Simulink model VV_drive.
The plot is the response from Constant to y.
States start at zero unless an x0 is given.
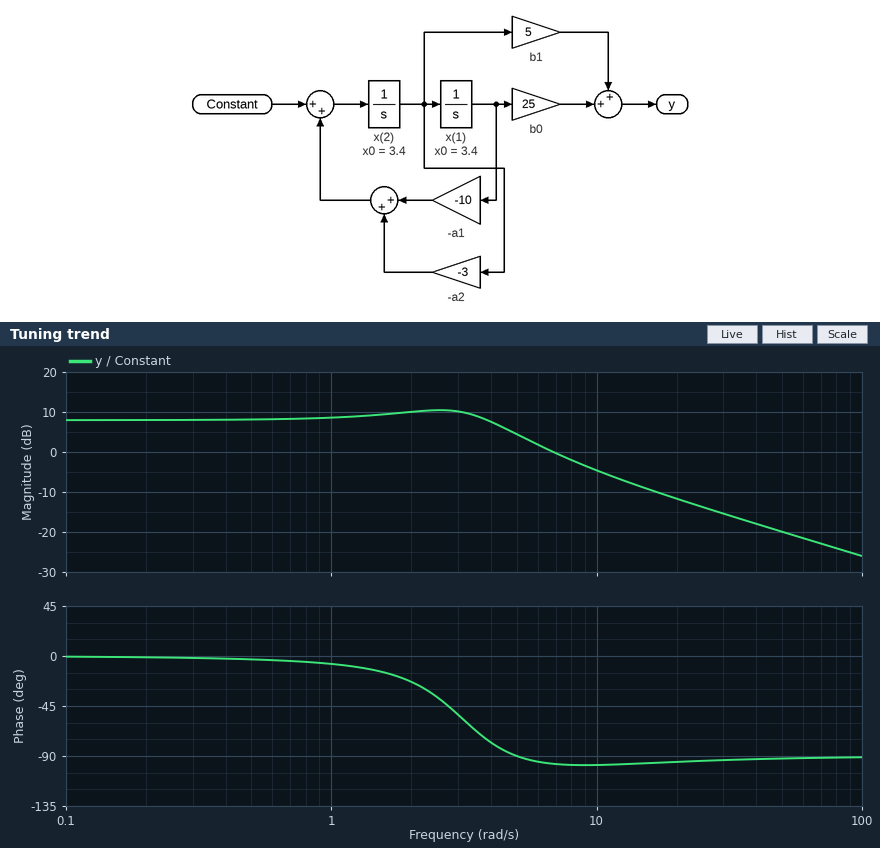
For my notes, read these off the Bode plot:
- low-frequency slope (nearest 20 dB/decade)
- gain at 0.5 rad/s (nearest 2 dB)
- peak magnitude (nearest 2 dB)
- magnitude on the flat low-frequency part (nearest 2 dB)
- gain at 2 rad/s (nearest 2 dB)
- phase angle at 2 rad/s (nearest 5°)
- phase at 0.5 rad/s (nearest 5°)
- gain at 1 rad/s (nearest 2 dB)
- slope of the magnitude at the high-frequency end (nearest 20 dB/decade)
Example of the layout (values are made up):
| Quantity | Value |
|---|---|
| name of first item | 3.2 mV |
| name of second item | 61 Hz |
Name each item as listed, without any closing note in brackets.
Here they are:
| Quantity | Value |
|---|---|
| low-frequency slope | 0 dB/decade |
| gain at 0.5 rad/s | 8 dB |
| peak magnitude | 10 dB |
| magnitude on the flat low-frequency part | 8 dB |
| gain at 2 rad/s | 10 dB |
| phase angle at 2 rad/s | -25° |
| phase at 0.5 rad/s | -5° |
| gain at 1 rad/s | 8 dB |
| slope of the magnitude at the high-frequency end | -20 dB/decade |
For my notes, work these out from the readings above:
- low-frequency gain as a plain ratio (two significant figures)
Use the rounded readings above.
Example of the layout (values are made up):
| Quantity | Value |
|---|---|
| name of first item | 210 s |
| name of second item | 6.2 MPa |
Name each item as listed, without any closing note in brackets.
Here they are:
| Quantity | Value |
|---|---|
| low-frequency gain as a plain ratio | 2.5 |
